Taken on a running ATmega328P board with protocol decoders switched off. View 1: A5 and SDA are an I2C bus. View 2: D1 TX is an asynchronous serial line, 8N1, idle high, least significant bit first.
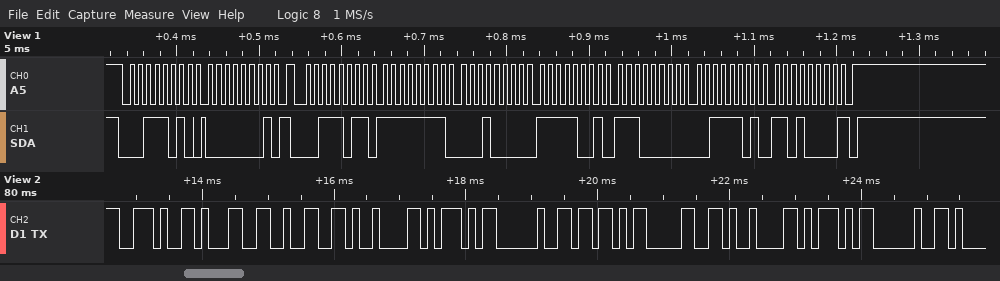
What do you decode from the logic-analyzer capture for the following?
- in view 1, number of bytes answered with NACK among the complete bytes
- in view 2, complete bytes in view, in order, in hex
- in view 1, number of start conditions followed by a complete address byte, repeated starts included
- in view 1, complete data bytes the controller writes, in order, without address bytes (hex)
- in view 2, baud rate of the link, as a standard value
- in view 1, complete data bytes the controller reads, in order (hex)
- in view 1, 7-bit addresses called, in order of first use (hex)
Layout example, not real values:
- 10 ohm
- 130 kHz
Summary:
- 1
- 2E 31 32 09 5D 20 5B 30 09 5D 20
- 2
- 01
- 9600 baud
- FF 10 F9 E0 3D D0
- 0x1D
